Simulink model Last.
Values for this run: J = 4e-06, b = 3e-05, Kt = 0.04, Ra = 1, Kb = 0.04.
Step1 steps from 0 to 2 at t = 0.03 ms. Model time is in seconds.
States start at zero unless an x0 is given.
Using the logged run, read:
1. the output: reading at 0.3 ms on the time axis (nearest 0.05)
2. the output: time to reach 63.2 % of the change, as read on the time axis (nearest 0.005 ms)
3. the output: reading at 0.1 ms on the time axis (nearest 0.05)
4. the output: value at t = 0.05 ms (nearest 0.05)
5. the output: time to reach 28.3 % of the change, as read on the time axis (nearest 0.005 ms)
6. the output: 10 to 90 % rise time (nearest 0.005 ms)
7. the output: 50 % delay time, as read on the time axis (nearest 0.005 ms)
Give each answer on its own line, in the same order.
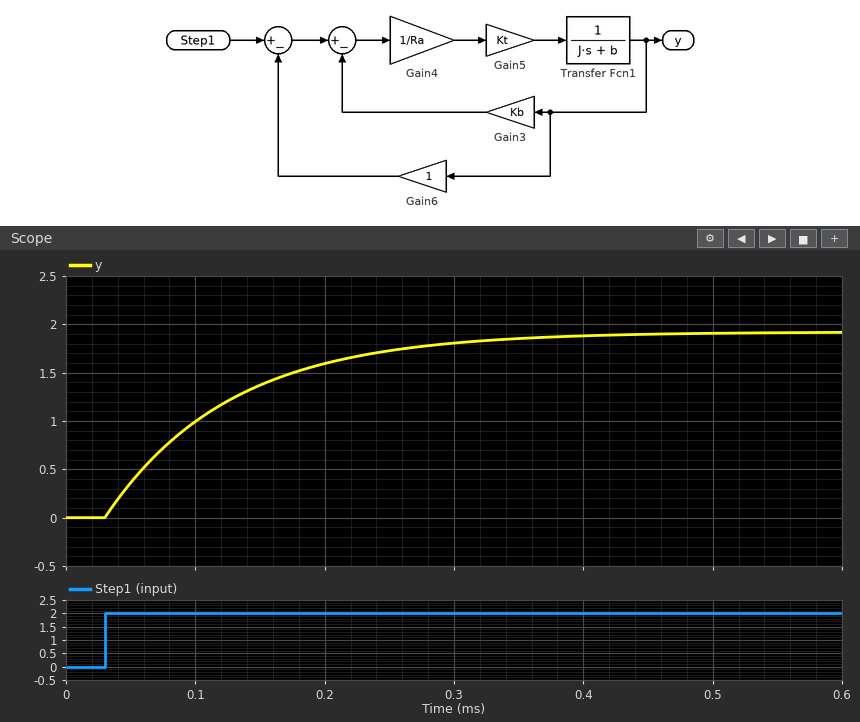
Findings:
1.80
0.125 ms
1.00
0.35
0.060 ms
0.210 ms
0.095 ms
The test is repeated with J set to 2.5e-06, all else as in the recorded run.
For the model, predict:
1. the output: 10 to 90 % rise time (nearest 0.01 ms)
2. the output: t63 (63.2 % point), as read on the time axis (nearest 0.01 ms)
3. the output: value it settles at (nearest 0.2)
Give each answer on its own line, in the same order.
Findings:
0.13 ms
0.09 ms
2.0
